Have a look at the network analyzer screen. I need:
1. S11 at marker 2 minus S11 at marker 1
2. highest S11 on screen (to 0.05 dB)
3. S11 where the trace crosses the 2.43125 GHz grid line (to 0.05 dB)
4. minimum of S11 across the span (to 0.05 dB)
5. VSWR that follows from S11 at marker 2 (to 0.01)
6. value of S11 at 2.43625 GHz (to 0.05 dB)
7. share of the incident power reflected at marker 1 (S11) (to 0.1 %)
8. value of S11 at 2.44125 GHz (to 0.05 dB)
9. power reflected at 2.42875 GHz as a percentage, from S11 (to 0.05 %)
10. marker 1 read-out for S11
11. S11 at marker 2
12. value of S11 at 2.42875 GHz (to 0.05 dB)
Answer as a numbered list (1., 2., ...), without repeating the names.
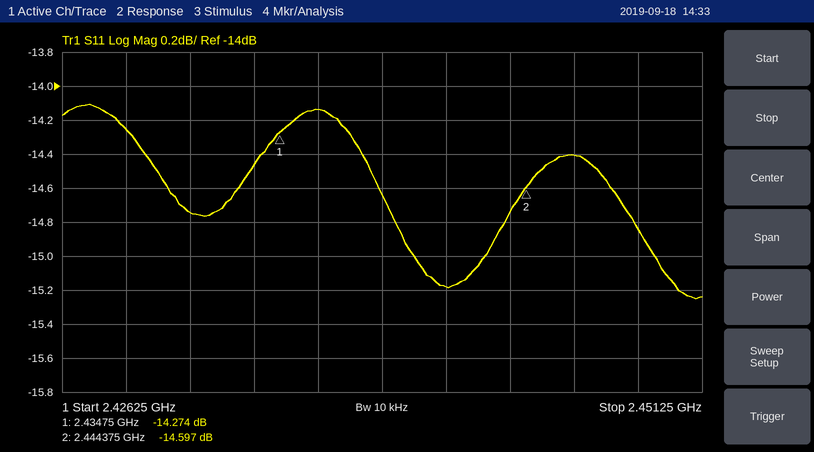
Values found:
1. -0.323 dB
2. -14.10 dB
3. -14.75 dB
4. -15.25 dB
5. 1.46
6. -14.15 dB
7. 3.7 %
8. -15.20 dB
9. 3.75 %
10. -14.274 dB
11. -14.597 dB
12. -14.25 dB
